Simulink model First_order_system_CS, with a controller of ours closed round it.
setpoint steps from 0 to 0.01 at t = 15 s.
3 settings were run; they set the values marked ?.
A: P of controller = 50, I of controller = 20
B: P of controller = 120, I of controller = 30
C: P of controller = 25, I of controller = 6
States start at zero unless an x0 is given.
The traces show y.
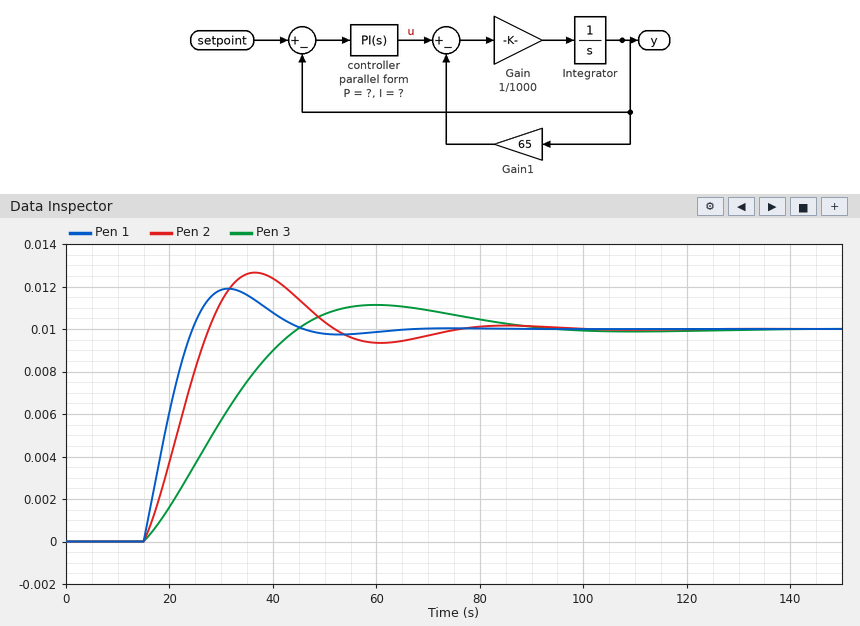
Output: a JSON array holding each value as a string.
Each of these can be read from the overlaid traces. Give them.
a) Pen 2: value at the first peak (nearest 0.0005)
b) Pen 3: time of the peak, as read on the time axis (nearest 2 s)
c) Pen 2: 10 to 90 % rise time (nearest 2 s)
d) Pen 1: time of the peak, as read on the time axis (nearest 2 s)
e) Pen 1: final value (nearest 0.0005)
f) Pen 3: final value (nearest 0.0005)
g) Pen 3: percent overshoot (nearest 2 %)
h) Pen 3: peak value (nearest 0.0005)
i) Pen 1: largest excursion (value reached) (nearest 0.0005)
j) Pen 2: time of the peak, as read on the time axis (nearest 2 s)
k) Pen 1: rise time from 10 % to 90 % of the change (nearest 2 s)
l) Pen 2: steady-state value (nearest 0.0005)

["0.0125", "60 s", "10 s", "32 s", "0.0100", "0.0100", "12 %", "0.0110", "0.0120", "36 s", "8 s", "0.0100"]
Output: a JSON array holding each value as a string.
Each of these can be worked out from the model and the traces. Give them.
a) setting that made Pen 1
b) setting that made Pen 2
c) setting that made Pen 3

["B", "A", "C"]
